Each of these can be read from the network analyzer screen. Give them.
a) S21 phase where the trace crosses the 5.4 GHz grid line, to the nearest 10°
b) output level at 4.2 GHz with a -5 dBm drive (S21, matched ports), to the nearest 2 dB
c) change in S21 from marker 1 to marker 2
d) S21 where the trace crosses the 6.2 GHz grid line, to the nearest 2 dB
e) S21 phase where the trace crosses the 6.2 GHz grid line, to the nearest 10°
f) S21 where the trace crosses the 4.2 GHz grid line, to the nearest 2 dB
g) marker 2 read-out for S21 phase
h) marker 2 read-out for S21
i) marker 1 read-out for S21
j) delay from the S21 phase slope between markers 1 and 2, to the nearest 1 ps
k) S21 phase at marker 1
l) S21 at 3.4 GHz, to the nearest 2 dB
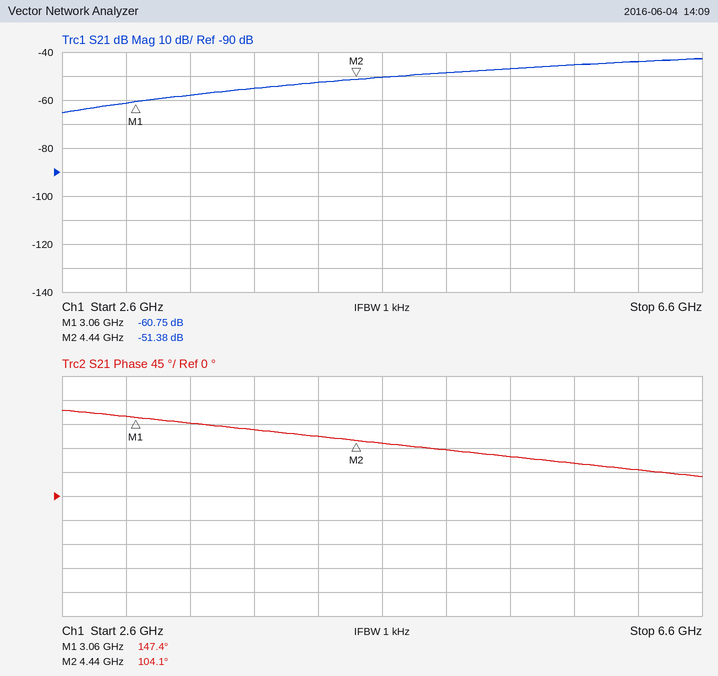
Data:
70°
-58 dBm
9.37 dB
-44 dB
50°
-52 dB
104.1°
-51.38 dB
-60.75 dB
87 ps
147.4°
-58 dB
